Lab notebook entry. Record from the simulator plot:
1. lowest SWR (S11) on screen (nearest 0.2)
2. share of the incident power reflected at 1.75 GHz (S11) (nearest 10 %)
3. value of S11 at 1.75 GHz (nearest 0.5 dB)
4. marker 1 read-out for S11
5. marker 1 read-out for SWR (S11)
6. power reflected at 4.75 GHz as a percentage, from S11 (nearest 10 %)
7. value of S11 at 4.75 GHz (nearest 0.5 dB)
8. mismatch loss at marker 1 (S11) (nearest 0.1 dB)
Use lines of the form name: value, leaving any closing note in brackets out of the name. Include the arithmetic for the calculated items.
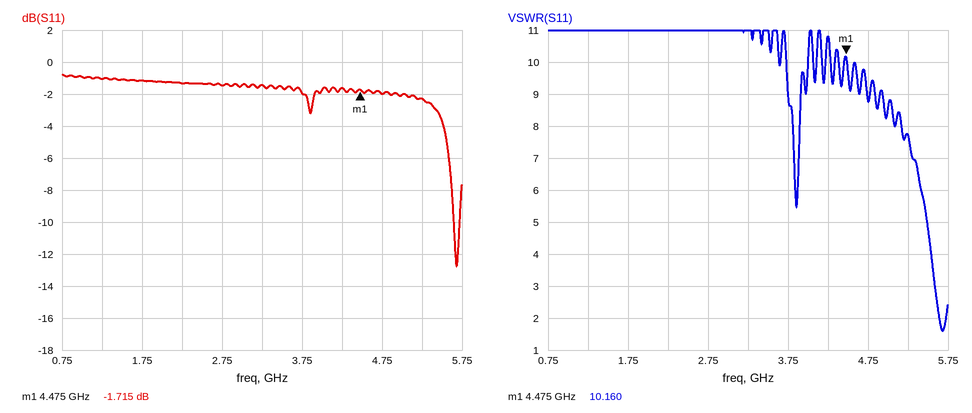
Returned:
lowest SWR (S11) on screen: 1.6
share of the incident power reflected at 1.75 GHz (S11): 10^(-1/10) ≈ 79.4 %, so 80 % to the nearest 10 %
value of S11 at 1.75 GHz: -1.0 dB
marker 1 read-out for S11: -1.715 dB
marker 1 read-out for SWR: 10.160
power reflected at 4.75 GHz as a percentage, from S11: 10^(-2/10) ≈ 63.1 %, so 60 % to the nearest 10 %
value of S11 at 4.75 GHz: -2.0 dB
mismatch loss at marker 1 (S11): −10 log10(1 − 10^(-1.715/10)) ≈ 4.9 dB
